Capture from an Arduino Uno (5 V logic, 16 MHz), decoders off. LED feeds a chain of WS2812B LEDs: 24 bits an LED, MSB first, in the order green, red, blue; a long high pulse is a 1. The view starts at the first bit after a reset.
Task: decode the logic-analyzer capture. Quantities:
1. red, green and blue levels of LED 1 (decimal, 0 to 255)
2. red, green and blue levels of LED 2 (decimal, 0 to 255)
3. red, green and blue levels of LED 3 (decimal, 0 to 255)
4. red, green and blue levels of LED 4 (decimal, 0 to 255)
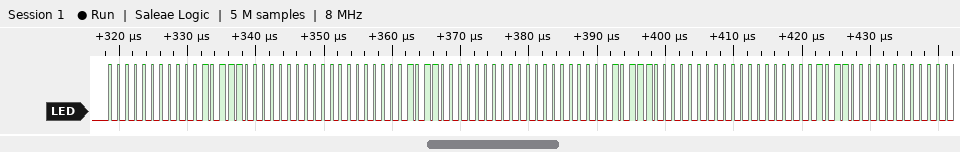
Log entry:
23, 0, 0
22, 0, 0
23, 0, 0
22, 0, 0
